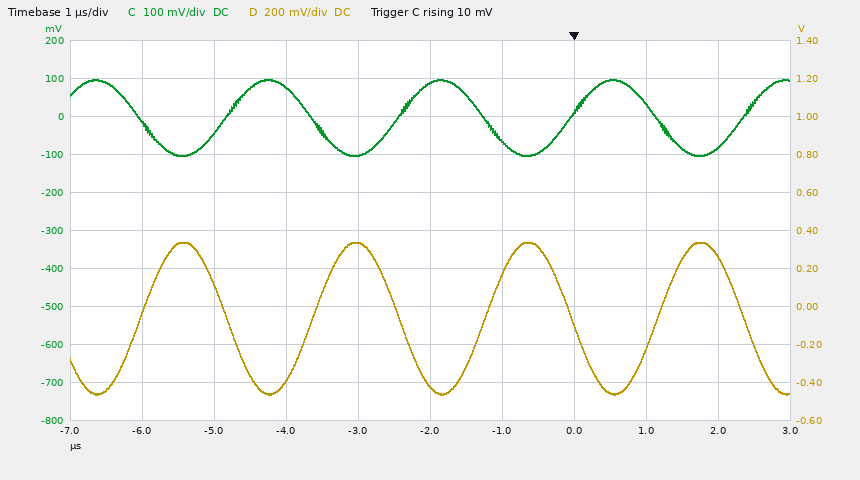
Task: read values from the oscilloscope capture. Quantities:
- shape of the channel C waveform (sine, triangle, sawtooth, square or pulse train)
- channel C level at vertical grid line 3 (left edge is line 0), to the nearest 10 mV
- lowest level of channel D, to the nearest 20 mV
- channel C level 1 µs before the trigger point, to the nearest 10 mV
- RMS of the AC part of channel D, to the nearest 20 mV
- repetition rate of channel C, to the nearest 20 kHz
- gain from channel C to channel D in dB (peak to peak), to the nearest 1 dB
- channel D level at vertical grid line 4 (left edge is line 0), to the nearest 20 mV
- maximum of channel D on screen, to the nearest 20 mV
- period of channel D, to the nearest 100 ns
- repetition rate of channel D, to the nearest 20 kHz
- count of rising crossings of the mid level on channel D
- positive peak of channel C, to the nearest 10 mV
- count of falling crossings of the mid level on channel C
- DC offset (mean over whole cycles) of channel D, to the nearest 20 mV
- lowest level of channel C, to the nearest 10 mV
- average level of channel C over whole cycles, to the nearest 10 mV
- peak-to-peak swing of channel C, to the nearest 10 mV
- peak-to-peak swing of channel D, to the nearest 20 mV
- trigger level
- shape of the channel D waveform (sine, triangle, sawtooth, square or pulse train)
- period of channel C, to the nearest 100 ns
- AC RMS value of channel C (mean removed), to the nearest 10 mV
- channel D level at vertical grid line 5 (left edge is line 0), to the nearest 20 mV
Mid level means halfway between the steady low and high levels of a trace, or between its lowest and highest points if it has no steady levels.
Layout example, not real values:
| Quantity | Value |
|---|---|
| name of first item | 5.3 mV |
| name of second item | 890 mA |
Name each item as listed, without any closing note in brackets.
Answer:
| Quantity | Value |
|---|---|
| shape of the channel C waveform | sine |
| channel C level at vertical grid line 3 (left edge is line 0), to the nearest 10 mV | 80 mV |
| lowest level of channel D, to the nearest 20 mV | -460 mV |
| channel C level 1 µs before the trigger point, to the nearest 10 mV | -60 mV |
| RMS of the AC part of channel D, to the nearest 20 mV | 280 mV |
| repetition rate of channel C, to the nearest 20 kHz | 420 kHz |
| gain from channel C to channel D in dB (peak to peak), to the nearest 1 dB | 12 dB |
| channel D level at vertical grid line 4 (left edge is line 0), to the nearest 20 mV | 340 mV |
| maximum of channel D on screen, to the nearest 20 mV | 340 mV |
| period of channel D, to the nearest 100 ns | 2.4 µs |
| repetition rate of channel D, to the nearest 20 kHz | 420 kHz |
| count of rising crossings of the mid level on channel D | 4 |
| positive peak of channel C, to the nearest 10 mV | 100 mV |
| count of falling crossings of the mid level on channel C | 4 |
| DC offset (mean over whole cycles) of channel D, to the nearest 20 mV | -60 mV |
| lowest level of channel C, to the nearest 10 mV | -100 mV |
| average level of channel C over whole cycles, to the nearest 10 mV | 0 mV |
| peak-to-peak swing of channel C, to the nearest 10 mV | 200 mV |
| peak-to-peak swing of channel D, to the nearest 20 mV | 800 mV |
| trigger level | 10 mV |
| shape of the channel D waveform | sine |
| period of channel C, to the nearest 100 ns | 2.4 µs |
| AC RMS value of channel C (mean removed), to the nearest 10 mV | 70 mV |
| channel D level at vertical grid line 5 (left edge is line 0), to the nearest 20 mV | -420 mV |
